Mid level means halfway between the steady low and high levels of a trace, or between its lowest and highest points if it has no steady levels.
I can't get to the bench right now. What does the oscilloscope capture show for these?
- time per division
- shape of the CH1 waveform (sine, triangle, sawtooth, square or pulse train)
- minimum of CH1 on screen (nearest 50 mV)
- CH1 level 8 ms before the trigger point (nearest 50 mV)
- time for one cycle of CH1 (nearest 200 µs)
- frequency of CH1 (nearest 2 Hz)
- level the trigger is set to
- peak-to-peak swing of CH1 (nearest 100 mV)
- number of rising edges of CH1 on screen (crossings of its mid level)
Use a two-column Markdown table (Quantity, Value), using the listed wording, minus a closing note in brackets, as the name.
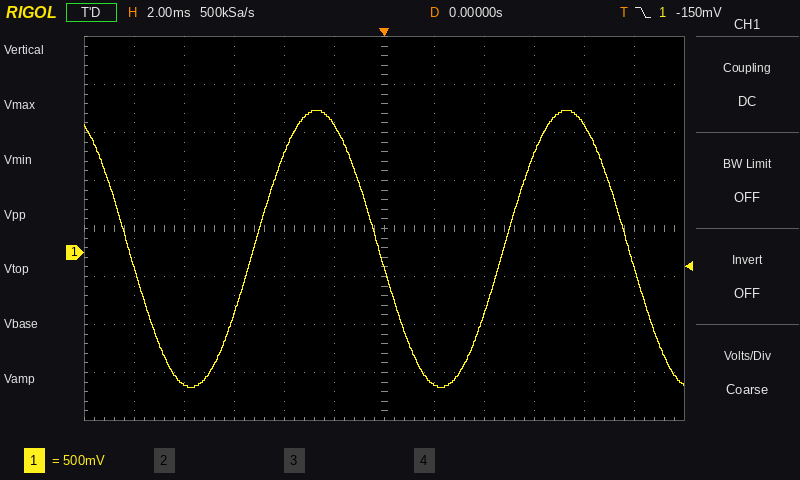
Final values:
| Quantity | Value |
|---|---|
| time per division | 2 ms |
| shape of the CH1 waveform | sine |
| minimum of CH1 on screen | -1.40 V |
| CH1 level 8 ms before the trigger point | -1.35 V |
| time for one cycle of CH1 | 10.0 ms |
| frequency of CH1 | 100 Hz |
| level the trigger is set to | -150 mV |
| peak-to-peak swing of CH1 | 2.90 V |
| number of rising edges of CH1 on screen | 2 |
